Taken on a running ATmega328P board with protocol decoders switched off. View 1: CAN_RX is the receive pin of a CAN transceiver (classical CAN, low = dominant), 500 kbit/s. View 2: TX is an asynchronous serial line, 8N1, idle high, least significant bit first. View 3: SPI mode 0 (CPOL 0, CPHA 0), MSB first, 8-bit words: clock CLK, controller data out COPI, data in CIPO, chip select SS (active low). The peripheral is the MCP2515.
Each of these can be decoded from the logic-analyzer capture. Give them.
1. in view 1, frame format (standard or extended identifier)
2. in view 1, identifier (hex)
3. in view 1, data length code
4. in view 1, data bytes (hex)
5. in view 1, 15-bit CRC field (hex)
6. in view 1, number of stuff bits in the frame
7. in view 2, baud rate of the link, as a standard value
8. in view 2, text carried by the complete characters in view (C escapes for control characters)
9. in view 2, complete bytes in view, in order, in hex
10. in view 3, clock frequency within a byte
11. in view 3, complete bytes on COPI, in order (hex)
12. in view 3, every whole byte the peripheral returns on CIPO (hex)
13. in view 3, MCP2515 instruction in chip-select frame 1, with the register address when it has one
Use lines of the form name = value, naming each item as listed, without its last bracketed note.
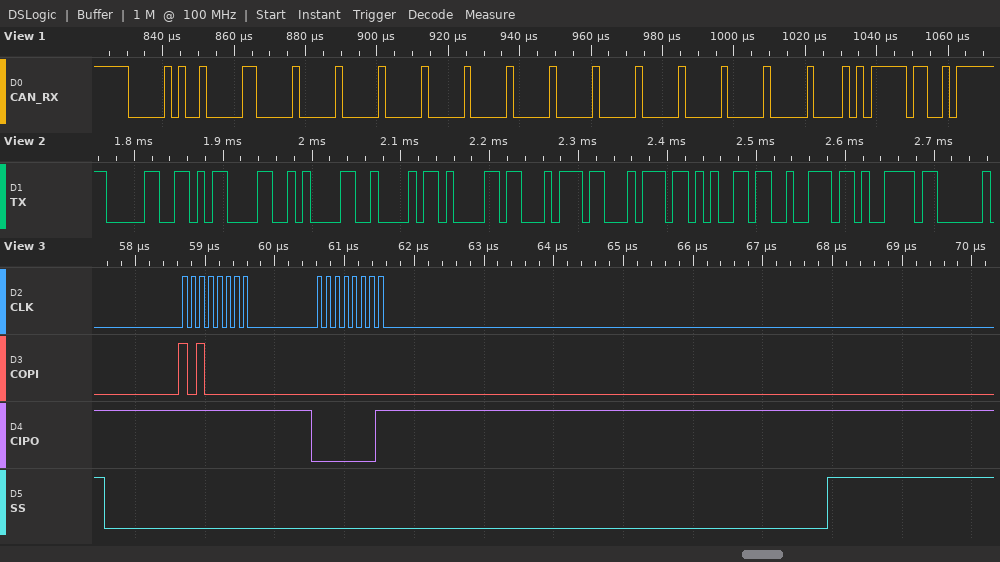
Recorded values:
in view 1, frame format = standard
in view 1, identifier = 0x024
in view 1, data length code = 8
in view 1, data bytes = 00 00 00 00 00 00 00 00
in view 1, 15-bit CRC field = 0x15FC
in view 1, number of stuff bits in the frame = 16
in view 2, baud rate of the link, as a standard value = 115200 baud
in view 2, text carried by the complete characters in view = "0\r\nBattery"
in view 2, complete bytes in view, in order, in hex = 0x30 0x0D 0x0A 0x42 0x61 0x74 0x74 0x65 0x72 0x79
in view 3, clock frequency within a byte = 8 MHz
in view 3, complete bytes on COPI, in order = A0 00
in view 3, every whole byte the peripheral returns on CIPO = FF 01
in view 3, MCP2515 instruction in chip-select frame 1, with the register address when it has one = READ STATUS
